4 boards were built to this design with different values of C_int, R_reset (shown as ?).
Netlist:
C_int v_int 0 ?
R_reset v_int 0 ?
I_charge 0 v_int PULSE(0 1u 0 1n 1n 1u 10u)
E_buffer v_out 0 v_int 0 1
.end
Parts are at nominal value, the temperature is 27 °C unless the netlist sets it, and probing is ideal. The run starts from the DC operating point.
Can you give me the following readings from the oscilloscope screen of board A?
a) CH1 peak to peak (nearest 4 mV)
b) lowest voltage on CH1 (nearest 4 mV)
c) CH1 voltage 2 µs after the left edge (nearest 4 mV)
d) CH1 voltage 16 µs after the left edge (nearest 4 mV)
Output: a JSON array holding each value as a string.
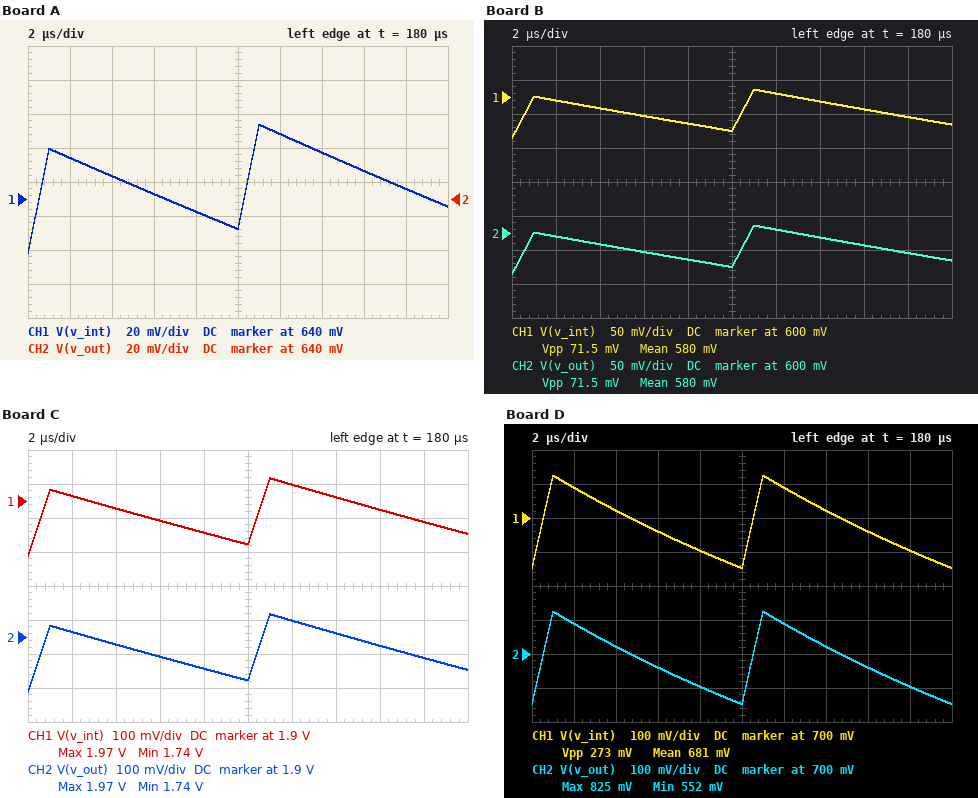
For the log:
["76 mV", "608 mV", "664 mV", "656 mV"]
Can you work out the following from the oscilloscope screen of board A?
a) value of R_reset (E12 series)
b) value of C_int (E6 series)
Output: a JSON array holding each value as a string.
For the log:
["8.2 MΩ", "15 pF"]
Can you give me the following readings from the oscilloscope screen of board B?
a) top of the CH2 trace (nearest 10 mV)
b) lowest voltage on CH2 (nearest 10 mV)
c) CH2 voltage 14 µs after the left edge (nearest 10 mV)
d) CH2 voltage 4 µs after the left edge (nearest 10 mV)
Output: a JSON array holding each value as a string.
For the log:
["610 mV", "540 mV", "590 mV", "580 mV"]
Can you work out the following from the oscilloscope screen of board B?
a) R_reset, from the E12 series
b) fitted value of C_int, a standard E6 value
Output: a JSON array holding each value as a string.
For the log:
["6.8 MΩ", "15 pF"]
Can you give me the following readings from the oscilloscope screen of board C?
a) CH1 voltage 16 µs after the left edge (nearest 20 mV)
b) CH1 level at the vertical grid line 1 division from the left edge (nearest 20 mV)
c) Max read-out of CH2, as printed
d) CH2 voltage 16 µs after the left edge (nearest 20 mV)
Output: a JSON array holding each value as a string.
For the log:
["1.88 V", "1.92 V", "1.97 V", "1.88 V"]
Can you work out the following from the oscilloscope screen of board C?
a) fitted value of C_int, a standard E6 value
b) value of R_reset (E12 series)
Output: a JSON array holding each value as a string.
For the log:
["4.7 pF", "22 MΩ"]
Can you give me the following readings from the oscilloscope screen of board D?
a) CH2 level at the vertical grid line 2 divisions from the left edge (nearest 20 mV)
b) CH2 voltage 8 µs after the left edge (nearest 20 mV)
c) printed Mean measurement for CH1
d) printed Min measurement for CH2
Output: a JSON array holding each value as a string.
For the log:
["720 mV", "600 mV", "681 mV", "552 mV"]
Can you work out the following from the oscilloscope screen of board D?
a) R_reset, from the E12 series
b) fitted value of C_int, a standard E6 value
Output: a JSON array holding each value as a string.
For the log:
["6.8 MΩ", "3.3 pF"]
